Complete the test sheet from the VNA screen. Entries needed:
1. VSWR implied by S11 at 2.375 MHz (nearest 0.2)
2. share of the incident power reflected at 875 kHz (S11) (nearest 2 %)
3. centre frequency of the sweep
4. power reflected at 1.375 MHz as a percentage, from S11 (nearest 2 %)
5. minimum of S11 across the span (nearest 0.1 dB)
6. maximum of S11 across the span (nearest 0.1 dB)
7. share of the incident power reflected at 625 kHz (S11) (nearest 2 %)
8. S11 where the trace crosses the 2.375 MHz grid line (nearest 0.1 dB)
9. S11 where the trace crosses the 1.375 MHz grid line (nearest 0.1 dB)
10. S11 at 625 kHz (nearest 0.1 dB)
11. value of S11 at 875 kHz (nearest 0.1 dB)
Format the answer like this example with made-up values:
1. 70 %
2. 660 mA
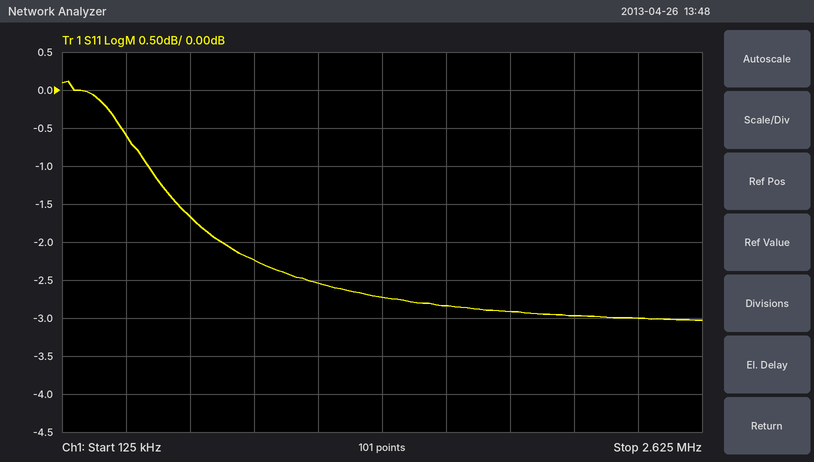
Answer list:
1. 5.8
2. 60 %
3. 1.375 MHz
4. 54 %
5. -3.0 dB
6. 0.1 dB
7. 68 %
8. -3.0 dB
9. -2.7 dB
10. -1.7 dB
11. -2.2 dB
